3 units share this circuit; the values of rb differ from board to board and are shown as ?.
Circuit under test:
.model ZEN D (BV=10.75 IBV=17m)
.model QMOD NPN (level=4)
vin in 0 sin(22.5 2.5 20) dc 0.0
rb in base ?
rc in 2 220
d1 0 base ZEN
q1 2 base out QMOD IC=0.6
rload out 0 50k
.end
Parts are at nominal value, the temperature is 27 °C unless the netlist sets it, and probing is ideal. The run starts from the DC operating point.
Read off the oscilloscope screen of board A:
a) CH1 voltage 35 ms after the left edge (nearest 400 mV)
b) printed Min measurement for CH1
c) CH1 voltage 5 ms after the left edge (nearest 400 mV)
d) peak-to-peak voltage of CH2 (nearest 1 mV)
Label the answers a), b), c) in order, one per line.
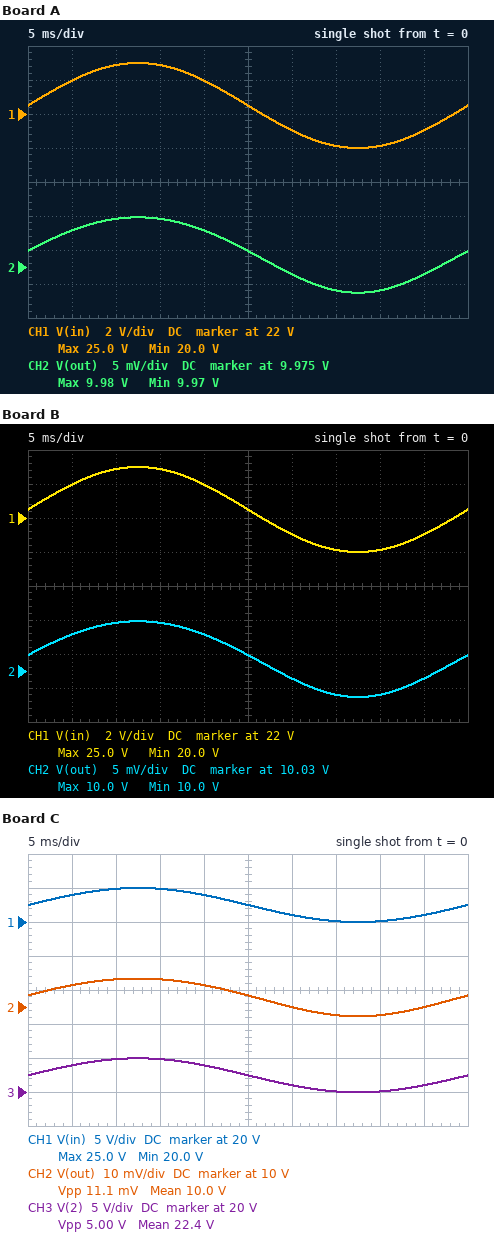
a) 20.0 V
b) 20.0 V
c) 24.0 V
d) 11 mV
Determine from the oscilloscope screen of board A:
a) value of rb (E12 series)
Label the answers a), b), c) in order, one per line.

a) 3.3 kΩ
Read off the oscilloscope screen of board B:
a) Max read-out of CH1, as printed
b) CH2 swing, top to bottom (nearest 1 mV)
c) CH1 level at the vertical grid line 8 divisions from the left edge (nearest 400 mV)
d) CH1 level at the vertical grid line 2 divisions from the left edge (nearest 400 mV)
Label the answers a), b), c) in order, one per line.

a) 25.0 V
b) 11 mV
c) 20.0 V
d) 24.8 V
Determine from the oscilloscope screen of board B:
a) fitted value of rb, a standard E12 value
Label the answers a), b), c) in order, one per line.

a) 390 Ω
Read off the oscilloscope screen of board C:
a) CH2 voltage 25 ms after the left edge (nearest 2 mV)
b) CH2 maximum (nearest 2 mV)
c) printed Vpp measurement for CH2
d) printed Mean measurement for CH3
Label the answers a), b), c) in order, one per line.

a) 10.004 V
b) 10.008 V
c) 11.1 mV
d) 22.4 V
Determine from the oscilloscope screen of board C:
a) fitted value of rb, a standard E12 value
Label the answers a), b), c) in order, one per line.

a) 1.2 kΩ
